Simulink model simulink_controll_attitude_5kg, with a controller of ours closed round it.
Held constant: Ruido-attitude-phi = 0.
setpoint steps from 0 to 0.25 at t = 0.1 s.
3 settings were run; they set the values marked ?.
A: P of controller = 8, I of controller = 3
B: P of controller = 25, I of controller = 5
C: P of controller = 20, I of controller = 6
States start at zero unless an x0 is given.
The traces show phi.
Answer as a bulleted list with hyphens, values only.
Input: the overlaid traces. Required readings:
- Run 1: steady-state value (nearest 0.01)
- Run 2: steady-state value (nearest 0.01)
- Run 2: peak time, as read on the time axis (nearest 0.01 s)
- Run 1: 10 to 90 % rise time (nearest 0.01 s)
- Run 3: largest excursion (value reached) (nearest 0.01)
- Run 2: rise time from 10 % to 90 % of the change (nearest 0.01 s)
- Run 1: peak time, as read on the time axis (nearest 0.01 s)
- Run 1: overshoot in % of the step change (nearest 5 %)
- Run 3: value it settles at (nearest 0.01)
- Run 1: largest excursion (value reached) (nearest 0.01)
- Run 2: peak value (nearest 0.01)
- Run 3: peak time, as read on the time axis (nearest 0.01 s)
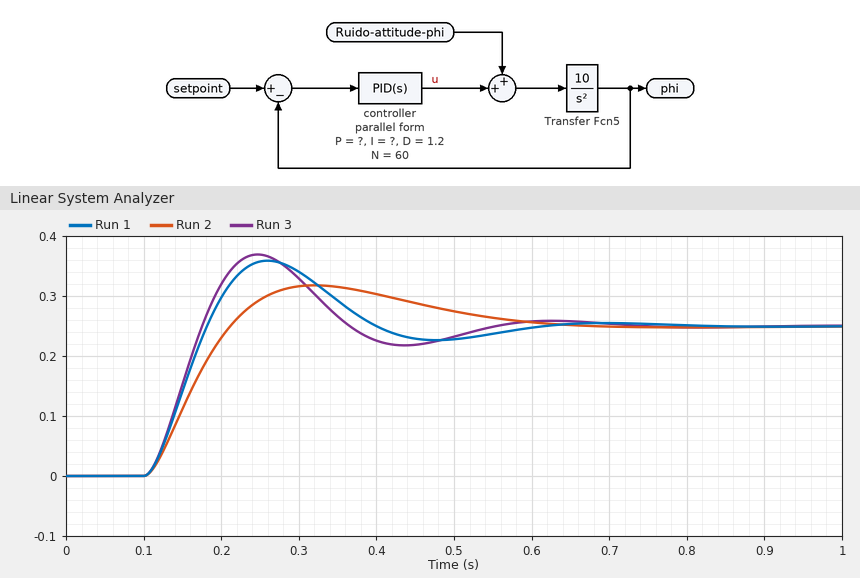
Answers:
- 0.25
- 0.25
- 0.32 s
- 0.06 s
- 0.37
- 0.08 s
- 0.26 s
- 45 %
- 0.25
- 0.36
- 0.32
- 0.25 s
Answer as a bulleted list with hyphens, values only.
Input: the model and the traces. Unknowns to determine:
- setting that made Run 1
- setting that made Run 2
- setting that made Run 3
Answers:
- C
- A
- B
